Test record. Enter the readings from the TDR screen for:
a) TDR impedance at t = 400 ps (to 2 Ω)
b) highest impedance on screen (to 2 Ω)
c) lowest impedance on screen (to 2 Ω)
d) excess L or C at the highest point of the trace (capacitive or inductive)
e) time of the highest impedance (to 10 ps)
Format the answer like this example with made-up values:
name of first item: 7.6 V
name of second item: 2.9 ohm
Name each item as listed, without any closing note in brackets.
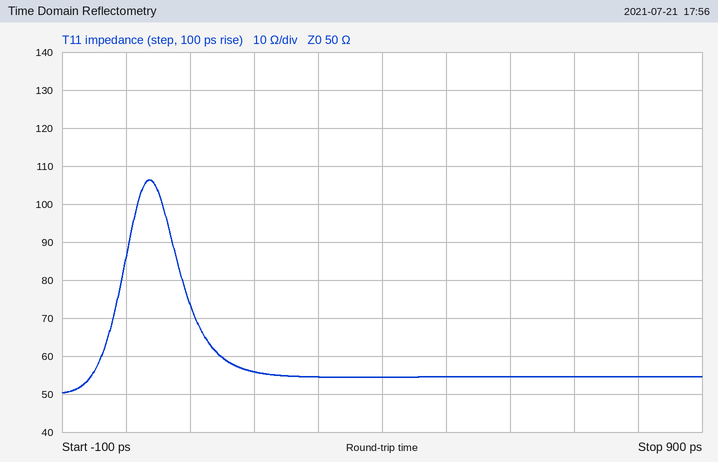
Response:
TDR impedance at t = 400 ps: 54 Ω
highest impedance on screen: 106 Ω
lowest impedance on screen: 50 Ω
excess L or C at the highest point of the trace: inductive
time of the highest impedance: 40 ps
